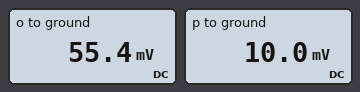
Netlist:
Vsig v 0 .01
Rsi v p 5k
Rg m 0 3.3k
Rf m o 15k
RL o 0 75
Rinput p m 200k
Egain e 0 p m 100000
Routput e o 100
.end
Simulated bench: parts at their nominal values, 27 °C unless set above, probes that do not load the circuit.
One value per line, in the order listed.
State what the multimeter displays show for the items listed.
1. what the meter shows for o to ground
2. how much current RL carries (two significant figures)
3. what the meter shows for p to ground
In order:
55.4 mV
740 µA
10.0 mV
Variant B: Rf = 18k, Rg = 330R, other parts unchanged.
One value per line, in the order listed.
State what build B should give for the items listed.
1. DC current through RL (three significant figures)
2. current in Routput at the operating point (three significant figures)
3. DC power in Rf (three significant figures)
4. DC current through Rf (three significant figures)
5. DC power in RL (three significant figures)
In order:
7.40 mA
7.43 mA
16.5 µW
30.3 µA
4.10 mW
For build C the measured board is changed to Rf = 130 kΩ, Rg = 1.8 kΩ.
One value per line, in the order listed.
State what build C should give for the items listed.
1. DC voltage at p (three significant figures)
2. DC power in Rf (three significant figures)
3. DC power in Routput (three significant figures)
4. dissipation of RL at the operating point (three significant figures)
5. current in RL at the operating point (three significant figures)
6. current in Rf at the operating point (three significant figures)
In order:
10.0 mV
4.00 µW
9.51 mW
7.12 mW
9.75 mA
5.55 µA
